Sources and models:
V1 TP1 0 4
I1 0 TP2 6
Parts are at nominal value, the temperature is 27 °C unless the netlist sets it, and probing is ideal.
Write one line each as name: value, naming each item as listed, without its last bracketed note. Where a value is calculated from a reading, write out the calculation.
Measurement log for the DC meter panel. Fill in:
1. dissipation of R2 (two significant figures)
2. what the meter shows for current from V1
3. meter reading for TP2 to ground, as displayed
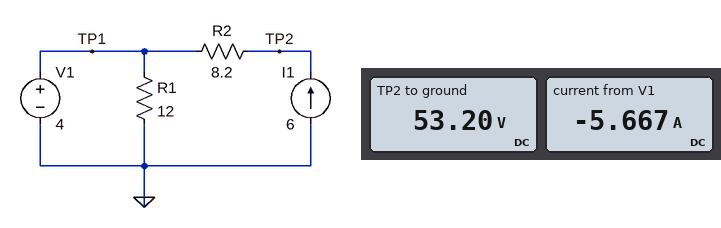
dissipation of R2: (53.2 V - 4 V)^2 / 8.2 Ω = 300 W
what the meter shows for current from V1: -5.667 A
meter reading for TP2 to ground, as displayed: 53.20 V
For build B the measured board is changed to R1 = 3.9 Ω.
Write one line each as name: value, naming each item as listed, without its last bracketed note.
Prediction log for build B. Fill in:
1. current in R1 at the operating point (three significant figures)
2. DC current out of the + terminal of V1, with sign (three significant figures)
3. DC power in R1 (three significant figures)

current in R1 at the operating point: 1.03 A
DC current out of the + terminal of V1, with sign: -4.97 A
DC power in R1: 4.10 W
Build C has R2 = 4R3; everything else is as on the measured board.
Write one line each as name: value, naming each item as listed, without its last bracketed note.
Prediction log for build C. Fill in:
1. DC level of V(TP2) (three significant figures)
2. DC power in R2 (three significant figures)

DC level of V(TP2): 29.8 V
DC power in R2: 155 W
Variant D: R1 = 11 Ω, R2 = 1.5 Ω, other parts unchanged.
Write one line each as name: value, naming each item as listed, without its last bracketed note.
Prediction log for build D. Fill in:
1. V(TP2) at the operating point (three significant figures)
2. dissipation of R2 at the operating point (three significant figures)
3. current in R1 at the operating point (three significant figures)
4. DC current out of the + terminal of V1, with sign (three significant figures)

V(TP2) at the operating point: 13.0 V
dissipation of R2 at the operating point: 54.0 W
current in R1 at the operating point: 364 mA
DC current out of the + terminal of V1, with sign: -5.64 A
